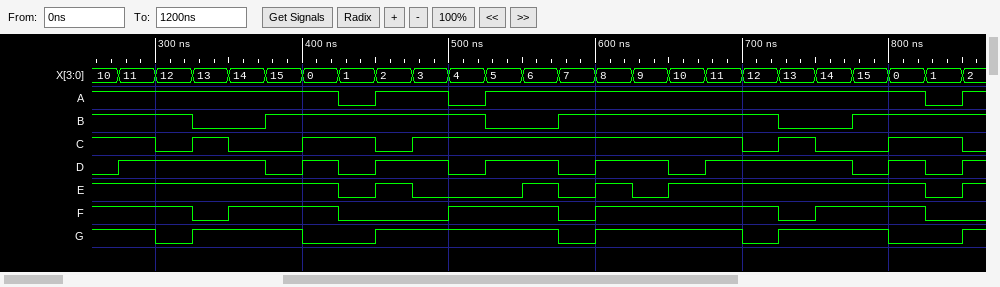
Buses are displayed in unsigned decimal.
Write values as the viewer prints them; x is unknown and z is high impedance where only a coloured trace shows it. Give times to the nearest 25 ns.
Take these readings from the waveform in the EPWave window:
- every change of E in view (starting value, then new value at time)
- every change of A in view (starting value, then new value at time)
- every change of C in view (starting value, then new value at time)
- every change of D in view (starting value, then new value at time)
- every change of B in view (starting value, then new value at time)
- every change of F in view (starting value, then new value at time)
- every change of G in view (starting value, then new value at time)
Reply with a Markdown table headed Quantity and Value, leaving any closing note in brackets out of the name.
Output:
| Quantity | Value |
|---|---|
| every change of E in view | 1, 0 at 425 ns, 1 at 450 ns, 0 at 475 ns, 1 at 550 ns, 0 at 575 ns, 1 at 600 ns, 0 at 625 ns, 1 at 650 ns, 0 at 825 ns, 1 at 850 ns |
| every change of A in view | 1, 0 at 425 ns, 1 at 450 ns, 0 at 500 ns, 1 at 525 ns, 0 at 825 ns, 1 at 850 ns |
| every change of C in view | 1, 0 at 300 ns, 1 at 325 ns, 0 at 350 ns, 1 at 400 ns, 0 at 450 ns, 1 at 475 ns, 0 at 700 ns, 1 at 725 ns, 0 at 750 ns, 1 at 800 ns, 0 at 850 ns |
| every change of D in view | 0, 1 at 275 ns, 0 at 375 ns, 1 at 400 ns, 0 at 425 ns, 1 at 450 ns, 0 at 500 ns, 1 at 525 ns, 0 at 575 ns, 1 at 600 ns, 0 at 650 ns, 1 at 675 ns, 0 at 775 ns, 1 at 800 ns, 0 at 825 ns, 1 at 850 ns |
| every change of B in view | 1, 0 at 325 ns, 1 at 375 ns, 0 at 525 ns, 1 at 575 ns, 0 at 725 ns, 1 at 775 ns |
| every change of F in view | 1, 0 at 325 ns, 1 at 350 ns, 0 at 425 ns, 1 at 500 ns, 0 at 575 ns, 1 at 600 ns, 0 at 725 ns, 1 at 750 ns, 0 at 825 ns |
| every change of G in view | 1, 0 at 300 ns, 1 at 325 ns, 0 at 400 ns, 1 at 450 ns, 0 at 575 ns, 1 at 600 ns, 0 at 700 ns, 1 at 725 ns, 0 at 800 ns, 1 at 850 ns |
